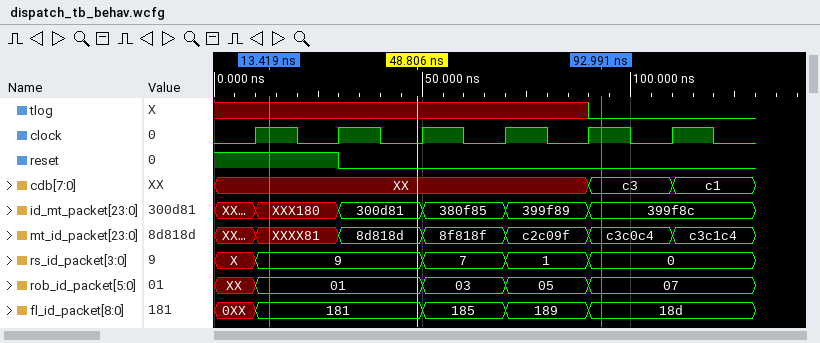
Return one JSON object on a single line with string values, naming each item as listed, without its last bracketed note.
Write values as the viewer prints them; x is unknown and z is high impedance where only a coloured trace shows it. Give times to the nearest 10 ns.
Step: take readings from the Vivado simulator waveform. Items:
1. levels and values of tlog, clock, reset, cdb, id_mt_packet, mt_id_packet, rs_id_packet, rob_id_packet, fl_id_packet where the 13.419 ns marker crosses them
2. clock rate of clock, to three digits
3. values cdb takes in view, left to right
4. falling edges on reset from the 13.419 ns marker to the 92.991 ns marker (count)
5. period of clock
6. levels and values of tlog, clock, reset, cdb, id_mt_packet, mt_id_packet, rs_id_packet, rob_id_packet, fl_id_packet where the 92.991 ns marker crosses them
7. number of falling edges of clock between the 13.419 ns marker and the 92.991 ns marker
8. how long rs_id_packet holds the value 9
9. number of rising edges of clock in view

{"levels and values of tlog, clock, reset, cdb, id_mt_packet, mt_id_packet, rs_id_packet, rob_id_packet, fl_id_packet where the 13.419 ns marker crosses them": "tlog=x, clock=1, reset=1, cdb=XX, id_mt_packet=XXX180, mt_id_packet=XXXX81, rs_id_packet=9, rob_id_packet=01, fl_id_packet=181", "clock rate of clock, to three digits": "50.0 MHz", "values cdb takes in view, left to right": "XX, c3, c1", "falling edges on reset from the 13.419 ns marker to the 92.991 ns marker": "1", "period of clock": "20 ns", "levels and values of tlog, clock, reset, cdb, id_mt_packet, mt_id_packet, rs_id_packet, rob_id_packet, fl_id_packet where the 92.991 ns marker crosses them": "tlog=0, clock=1, reset=0, cdb=c3, id_mt_packet=399f8c, mt_id_packet=c3c0c4, rs_id_packet=0, rob_id_packet=07, fl_id_packet=18d", "number of falling edges of clock between the 13.419 ns marker and the 92.991 ns marker": "4", "how long rs_id_packet holds the value 9": "40 ns", "number of rising edges of clock in view": "6"}
